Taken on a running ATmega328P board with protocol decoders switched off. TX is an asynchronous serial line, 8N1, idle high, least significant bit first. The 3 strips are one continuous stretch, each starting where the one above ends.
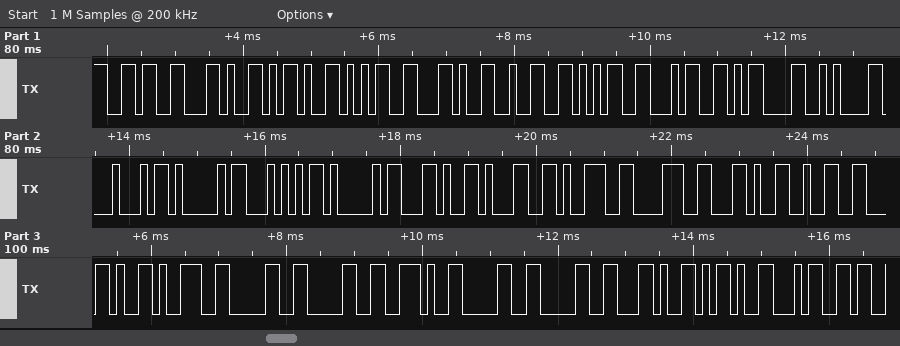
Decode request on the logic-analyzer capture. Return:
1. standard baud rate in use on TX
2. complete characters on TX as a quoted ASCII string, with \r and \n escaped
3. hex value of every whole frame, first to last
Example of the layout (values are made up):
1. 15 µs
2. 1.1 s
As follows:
1. 9600 baud
2. "6,-5,254\r\nDATA,198,2,900.00,-4"
3. 36 2C 2D 35 2C 32 35 34 0D 0A 44 41 54 41 2C 31 39 38 2C 32 2C 39 30 30 2E 30 30 2C 2D 34
